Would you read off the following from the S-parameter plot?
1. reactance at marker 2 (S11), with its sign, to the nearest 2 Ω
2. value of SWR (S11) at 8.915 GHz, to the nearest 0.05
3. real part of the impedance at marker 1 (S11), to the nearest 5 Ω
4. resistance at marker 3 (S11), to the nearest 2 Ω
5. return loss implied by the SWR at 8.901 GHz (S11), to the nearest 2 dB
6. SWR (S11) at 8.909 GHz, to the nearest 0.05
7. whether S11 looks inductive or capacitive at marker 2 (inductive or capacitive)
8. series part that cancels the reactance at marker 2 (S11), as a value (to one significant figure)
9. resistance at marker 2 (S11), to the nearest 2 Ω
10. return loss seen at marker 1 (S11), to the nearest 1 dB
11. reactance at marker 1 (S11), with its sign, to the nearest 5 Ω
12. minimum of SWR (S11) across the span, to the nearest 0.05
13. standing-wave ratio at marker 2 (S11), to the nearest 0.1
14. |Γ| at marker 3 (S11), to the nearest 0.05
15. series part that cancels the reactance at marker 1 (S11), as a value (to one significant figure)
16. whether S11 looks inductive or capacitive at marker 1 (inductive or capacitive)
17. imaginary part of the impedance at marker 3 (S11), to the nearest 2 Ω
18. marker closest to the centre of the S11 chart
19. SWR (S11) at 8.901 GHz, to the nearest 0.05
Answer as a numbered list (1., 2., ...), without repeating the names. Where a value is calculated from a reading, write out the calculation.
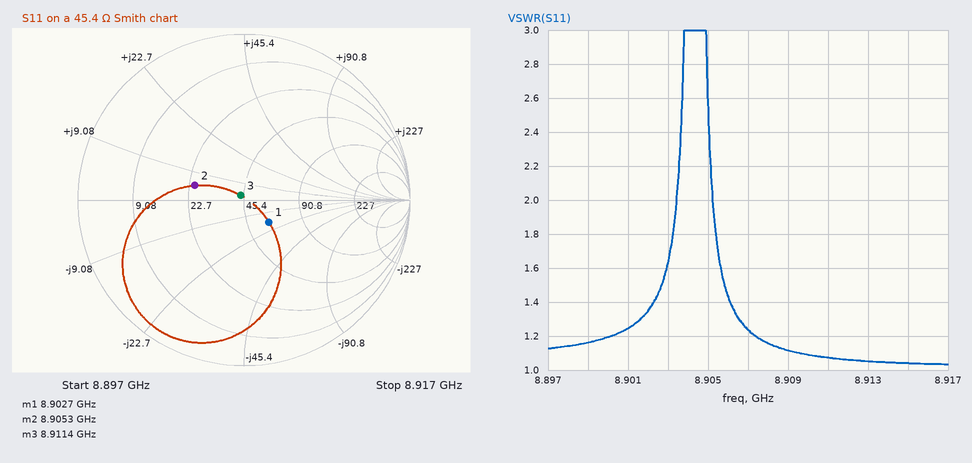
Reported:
1. +4 Ω
2. 1.05
3. 60 Ω
4. 44 Ω
5. −20 log10((1.25 − 1)/(1.25 + 1)) ≈ 19.1 dB, so 20 dB to the nearest 2 dB
6. 1.10
7. inductive
8. C = 1/(2π × 8.9053 GHz × 4 Ω) ≈ 4 pF
9. 24 Ω
10. 14 dB
11. -15 Ω
12. 1.05
13. 1.9
14. 0.05
15. L = 15 Ω/(2π × 8.9027 GHz) ≈ 268 pH, so 300 pH to one significant figure
16. capacitive
17. +2 Ω
18. marker 3
19. 1.25
